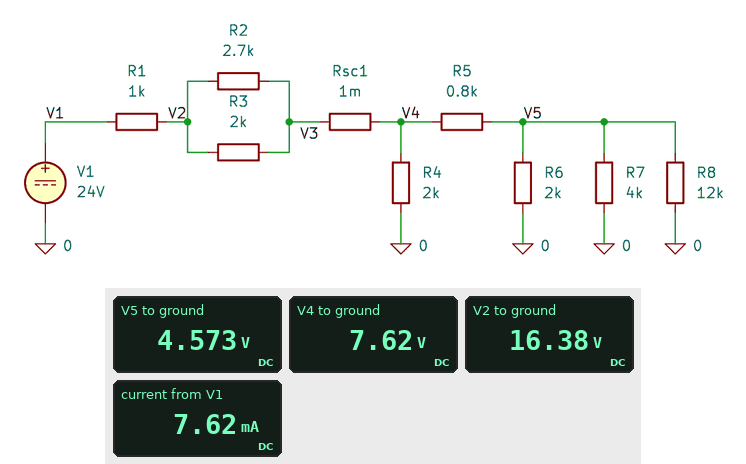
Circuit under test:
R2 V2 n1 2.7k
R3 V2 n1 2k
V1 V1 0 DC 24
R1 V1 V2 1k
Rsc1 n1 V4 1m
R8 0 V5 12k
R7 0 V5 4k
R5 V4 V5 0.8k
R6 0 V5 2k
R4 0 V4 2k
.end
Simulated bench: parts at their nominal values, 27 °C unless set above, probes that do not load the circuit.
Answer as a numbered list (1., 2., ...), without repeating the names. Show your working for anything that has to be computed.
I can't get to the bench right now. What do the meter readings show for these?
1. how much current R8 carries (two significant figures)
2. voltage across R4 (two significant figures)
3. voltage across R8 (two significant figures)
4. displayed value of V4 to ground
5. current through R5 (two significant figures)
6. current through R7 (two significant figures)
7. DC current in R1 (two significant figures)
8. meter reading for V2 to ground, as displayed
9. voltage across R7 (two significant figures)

1. (4.573 V) / 12 kΩ = 380 µA
2. 7.62 V = 7.6 V
3. 4.573 V = 4.6 V
4. 7.62 V
5. (7.62 V - 4.573 V) / 800 Ω = 3.8 mA
6. (4.573 V) / 4 kΩ = 1.1 mA
7. (24 V - 16.38 V) / 1 kΩ = 7.6 mA
8. 16.38 V
9. 4.573 V = 4.6 V
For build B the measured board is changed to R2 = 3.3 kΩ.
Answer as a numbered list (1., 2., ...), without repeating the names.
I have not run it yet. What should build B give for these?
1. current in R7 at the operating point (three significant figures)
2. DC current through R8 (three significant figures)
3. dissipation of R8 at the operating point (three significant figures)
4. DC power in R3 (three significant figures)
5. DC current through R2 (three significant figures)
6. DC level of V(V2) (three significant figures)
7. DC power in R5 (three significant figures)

1. 1.11 mA
2. 370 µA
3. 1.64 mW
4. 42.4 mW
5. 2.79 mA
6. 16.6 V
7. 10.9 mW
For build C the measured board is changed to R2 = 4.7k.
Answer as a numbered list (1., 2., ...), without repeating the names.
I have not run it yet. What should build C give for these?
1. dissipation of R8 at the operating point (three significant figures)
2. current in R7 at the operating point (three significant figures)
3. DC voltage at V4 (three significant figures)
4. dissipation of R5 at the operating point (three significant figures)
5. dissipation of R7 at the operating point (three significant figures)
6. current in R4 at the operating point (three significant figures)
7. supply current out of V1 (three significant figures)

1. 1.49 mW
2. 1.06 mA
3. 7.05 V
4. 9.95 mW
5. 4.48 mW
6. 3.53 mA
7. 7.05 mA
